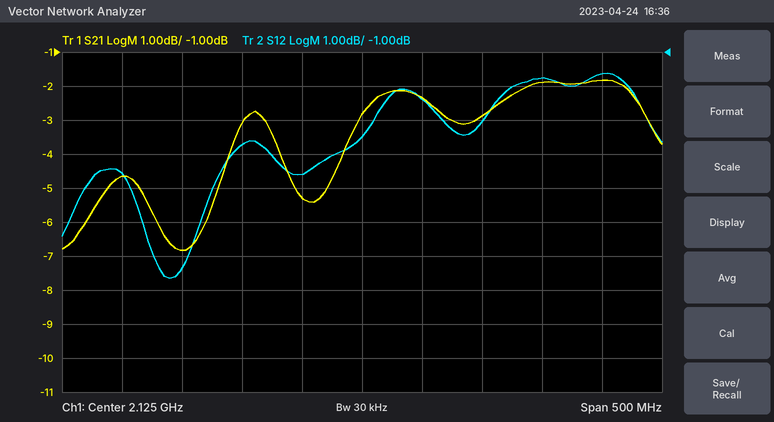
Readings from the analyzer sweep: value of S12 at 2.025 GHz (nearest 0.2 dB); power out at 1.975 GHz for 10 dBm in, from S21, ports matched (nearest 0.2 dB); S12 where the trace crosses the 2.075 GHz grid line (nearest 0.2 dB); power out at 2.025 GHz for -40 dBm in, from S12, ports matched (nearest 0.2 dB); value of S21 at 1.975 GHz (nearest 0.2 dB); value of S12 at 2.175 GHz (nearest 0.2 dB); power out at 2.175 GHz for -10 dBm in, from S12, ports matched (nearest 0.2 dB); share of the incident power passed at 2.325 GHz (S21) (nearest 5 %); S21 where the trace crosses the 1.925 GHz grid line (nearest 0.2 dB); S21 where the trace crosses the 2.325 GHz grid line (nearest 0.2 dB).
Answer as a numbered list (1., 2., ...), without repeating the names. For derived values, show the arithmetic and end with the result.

1. -3.8 dB
2. 10 dBm + (-6.8 dB) = 3.2 dBm
3. -4.6 dB
4. -40 dBm + (-3.8 dB) = -43.8 dBm
5. -6.8 dB
6. -2.4 dB
7. -10 dBm + (-2.4 dB) = -12.4 dBm
8. 10^(-1.8/10) ≈ 66.1 %, so 65 % to the nearest 5 %
9. -4.6 dB
10. -1.8 dB
